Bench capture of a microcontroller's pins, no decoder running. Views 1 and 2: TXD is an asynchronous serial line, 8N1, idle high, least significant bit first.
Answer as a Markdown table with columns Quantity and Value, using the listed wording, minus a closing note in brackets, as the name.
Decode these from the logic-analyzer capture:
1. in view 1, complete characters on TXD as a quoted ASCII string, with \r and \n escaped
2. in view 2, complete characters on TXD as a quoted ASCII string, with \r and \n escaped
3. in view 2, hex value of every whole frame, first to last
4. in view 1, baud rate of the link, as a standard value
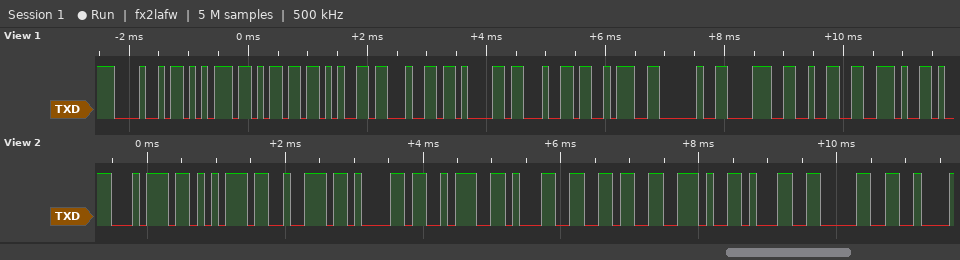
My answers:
| Quantity | Value |
|---|---|
| in view 1, complete characters on TXD as a quoted ASCII string, with \r and \n escaped | "Humedad: 82." |
| in view 2, complete characters on TXD as a quoted ASCII string, with \r and \n escaped | "tura:16.10" |
| in view 2, hex value of every whole frame, first to last | 74 75 72 61 3A 31 36 2E 31 30 |
| in view 1, baud rate of the link, as a standard value | 9600 baud |
